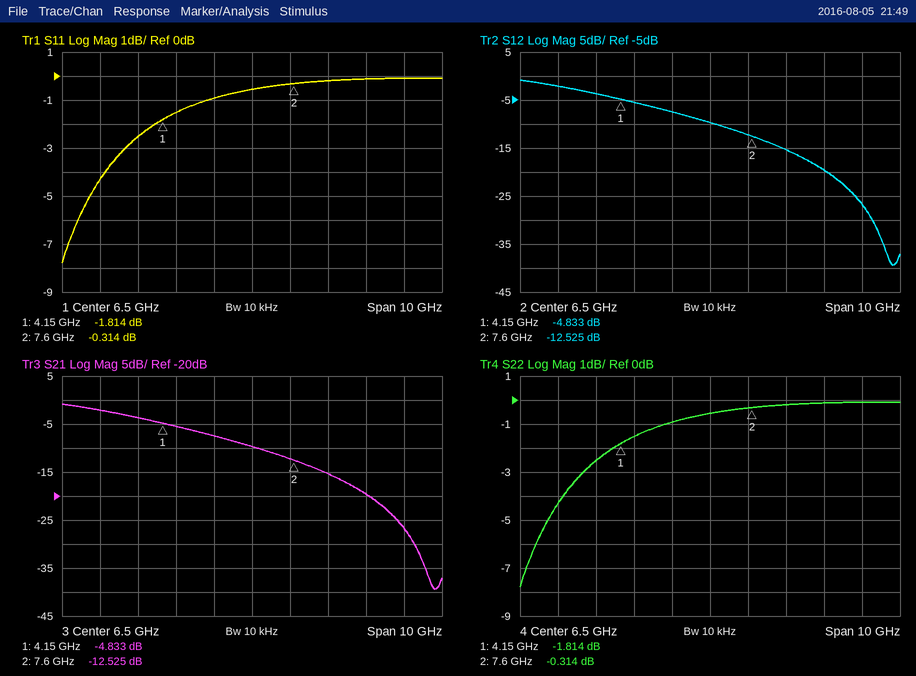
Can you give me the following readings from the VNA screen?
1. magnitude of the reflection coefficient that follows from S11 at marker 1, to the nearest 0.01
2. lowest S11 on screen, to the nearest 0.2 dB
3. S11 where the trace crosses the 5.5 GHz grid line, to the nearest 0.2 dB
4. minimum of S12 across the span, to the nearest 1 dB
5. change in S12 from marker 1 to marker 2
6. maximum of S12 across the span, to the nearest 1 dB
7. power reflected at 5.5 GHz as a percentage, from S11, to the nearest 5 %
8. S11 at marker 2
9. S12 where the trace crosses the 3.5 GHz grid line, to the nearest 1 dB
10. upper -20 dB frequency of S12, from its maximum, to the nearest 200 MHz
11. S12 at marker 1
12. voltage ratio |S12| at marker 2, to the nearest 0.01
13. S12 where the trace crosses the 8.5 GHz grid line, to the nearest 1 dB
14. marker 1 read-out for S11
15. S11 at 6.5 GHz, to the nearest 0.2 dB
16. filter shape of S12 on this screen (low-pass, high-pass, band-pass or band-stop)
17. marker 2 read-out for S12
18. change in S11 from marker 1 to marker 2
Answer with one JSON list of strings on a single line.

["0.81", "-7.8 dB", "-1.0 dB", "-39 dB", "-7.692 dB", "-1 dB", "80 %", "-0.314 dB", "-4 dB", "9.8 GHz", "-4.833 dB", "0.24", "-15 dB", "-1.814 dB", "-0.6 dB", "low-pass", "-12.525 dB", "1.500 dB"]
